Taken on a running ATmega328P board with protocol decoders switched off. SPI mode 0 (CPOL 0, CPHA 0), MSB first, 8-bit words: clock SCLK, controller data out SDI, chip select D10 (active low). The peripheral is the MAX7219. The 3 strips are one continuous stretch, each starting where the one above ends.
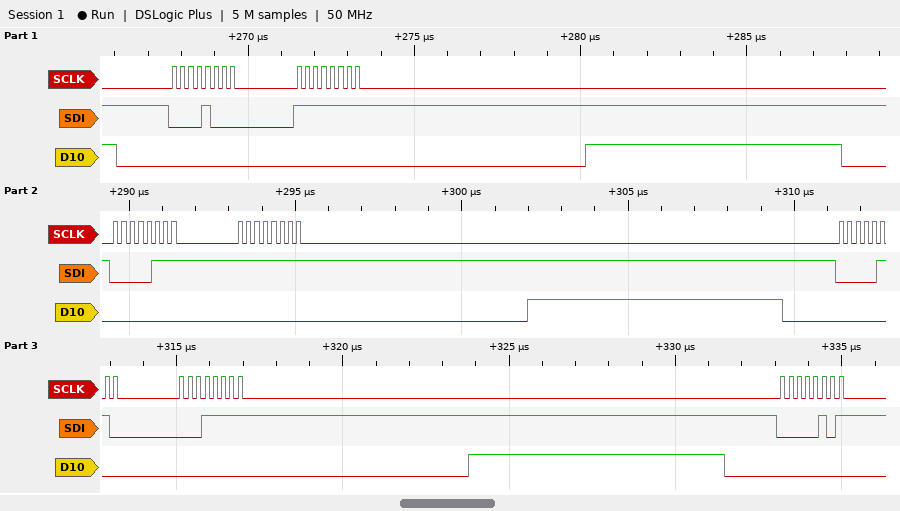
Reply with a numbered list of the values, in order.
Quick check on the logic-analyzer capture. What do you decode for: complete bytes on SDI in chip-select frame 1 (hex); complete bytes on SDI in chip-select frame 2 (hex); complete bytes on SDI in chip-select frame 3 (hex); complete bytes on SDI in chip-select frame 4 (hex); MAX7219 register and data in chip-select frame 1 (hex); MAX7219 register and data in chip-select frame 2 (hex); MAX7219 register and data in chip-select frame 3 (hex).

1. 08 FF
2. 07 FF
3. 06 1F
4. 05
5. register 0x8, data 0xFF
6. register 0x7, data 0xFF
7. register 0x6, data 0x1F
